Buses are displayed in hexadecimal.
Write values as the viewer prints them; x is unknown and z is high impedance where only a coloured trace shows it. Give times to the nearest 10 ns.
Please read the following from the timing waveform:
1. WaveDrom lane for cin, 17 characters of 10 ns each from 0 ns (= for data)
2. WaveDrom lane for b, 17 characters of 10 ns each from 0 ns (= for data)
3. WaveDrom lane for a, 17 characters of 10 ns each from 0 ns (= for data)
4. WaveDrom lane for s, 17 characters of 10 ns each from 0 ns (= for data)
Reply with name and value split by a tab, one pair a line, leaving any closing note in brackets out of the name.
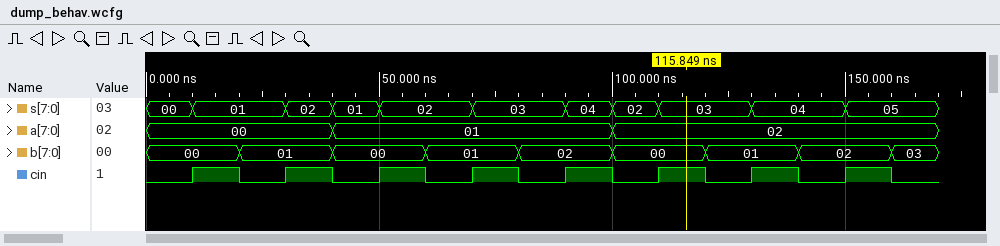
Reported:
WaveDrom lane for cin, 17 characters of 10 ns each from 0 ns	{name: 'cin', wave: '01010101010101010'}
WaveDrom lane for b, 17 characters of 10 ns each from 0 ns	{name: 'b', wave: '=.=.=.=.=.=.=.=.=', data: '00 01 00 01 02 00 01 02 03'}
WaveDrom lane for a, 17 characters of 10 ns each from 0 ns	{name: 'a', wave: '=...=.....=......', data: '00 01 02'}
WaveDrom lane for s, 17 characters of 10 ns each from 0 ns	{name: 's', wave: '==.===.=.===.=.=.', data: '00 01 02 01 02 03 04 02 03 04 05'}
